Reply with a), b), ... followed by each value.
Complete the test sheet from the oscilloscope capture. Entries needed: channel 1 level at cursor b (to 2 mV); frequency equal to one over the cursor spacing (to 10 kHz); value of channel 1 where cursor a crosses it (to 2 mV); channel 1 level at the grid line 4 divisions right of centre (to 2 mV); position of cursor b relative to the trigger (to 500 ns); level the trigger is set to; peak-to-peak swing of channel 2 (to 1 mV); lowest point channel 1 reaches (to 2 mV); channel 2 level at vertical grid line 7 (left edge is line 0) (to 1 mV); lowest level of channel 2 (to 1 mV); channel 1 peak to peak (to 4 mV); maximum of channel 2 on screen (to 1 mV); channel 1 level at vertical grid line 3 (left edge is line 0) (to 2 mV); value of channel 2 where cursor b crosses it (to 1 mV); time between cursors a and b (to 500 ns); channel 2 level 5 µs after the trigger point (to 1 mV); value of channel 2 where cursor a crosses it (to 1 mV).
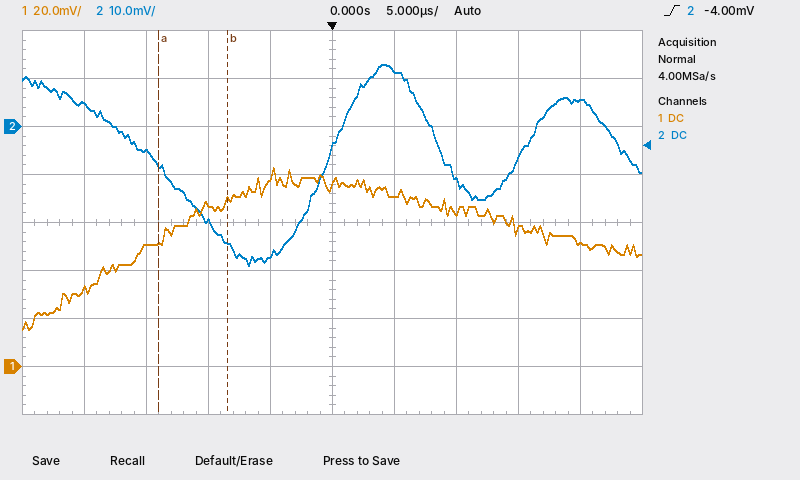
a) 68 mV
b) 180 kHz
c) 52 mV
d) 52 mV
e) -8.5 µs
f) -4.00 mV
g) 42 mV
h) 16 mV
i) -11 mV
j) -29 mV
k) 68 mV
l) 13 mV
m) 68 mV
n) -24 mV
o) 5.5 µs
p) 12 mV
q) -8 mV
